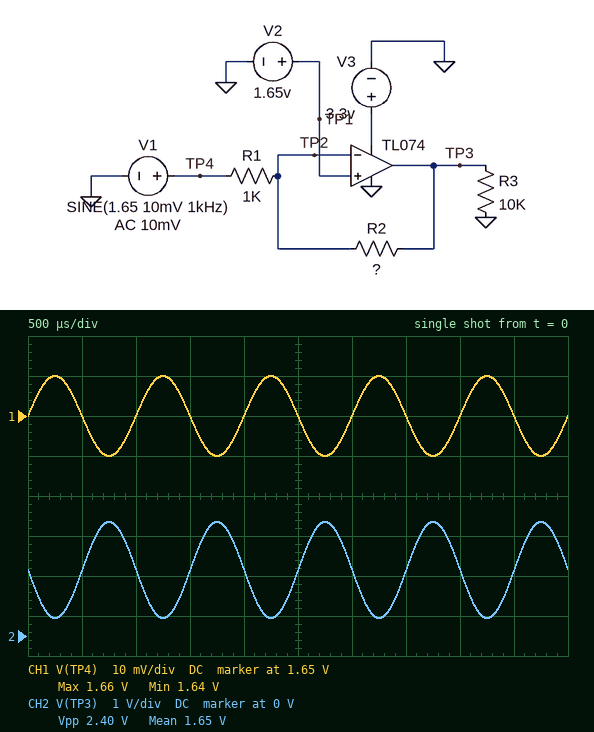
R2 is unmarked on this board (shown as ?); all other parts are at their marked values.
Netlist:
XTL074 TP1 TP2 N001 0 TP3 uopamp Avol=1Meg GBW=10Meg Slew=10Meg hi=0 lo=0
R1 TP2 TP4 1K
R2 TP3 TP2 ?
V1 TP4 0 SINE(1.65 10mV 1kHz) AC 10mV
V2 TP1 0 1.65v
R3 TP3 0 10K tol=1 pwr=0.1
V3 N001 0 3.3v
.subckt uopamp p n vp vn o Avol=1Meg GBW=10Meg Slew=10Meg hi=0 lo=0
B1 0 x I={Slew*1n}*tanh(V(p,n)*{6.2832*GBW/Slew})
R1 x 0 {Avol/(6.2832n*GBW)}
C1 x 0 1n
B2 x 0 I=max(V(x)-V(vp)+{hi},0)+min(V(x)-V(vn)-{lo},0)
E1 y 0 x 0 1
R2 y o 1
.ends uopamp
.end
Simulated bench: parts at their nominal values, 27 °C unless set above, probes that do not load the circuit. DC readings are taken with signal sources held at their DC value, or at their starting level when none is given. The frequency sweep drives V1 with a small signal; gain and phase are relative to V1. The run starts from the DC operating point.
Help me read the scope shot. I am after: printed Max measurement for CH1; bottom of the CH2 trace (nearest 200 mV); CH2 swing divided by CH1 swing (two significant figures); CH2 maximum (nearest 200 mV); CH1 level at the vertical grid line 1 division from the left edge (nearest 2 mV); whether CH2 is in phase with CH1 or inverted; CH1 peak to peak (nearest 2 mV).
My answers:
1.66 V
400 mV
120
2.8 V
1.650 V
inverted
20 mV
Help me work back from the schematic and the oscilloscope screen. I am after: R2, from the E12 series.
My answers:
120 kΩ
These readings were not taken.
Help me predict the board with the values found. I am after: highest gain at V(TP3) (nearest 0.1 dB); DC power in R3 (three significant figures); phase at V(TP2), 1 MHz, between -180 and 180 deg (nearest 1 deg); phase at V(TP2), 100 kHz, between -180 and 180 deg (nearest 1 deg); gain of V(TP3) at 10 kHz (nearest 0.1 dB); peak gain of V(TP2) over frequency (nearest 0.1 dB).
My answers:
41.6 dB
272 µW
5 deg
40 deg
41.5 dB
-0.1 dB
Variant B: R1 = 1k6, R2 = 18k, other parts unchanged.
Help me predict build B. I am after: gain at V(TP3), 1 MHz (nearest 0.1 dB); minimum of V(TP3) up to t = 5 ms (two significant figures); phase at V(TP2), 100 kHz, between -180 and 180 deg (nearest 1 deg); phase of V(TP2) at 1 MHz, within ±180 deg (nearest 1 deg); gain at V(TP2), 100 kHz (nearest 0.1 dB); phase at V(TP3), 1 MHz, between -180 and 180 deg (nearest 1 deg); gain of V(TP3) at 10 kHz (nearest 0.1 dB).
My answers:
17.0 dB
1.5 V
83 deg
39 deg
-19.0 dB
129 deg
21.0 dB
